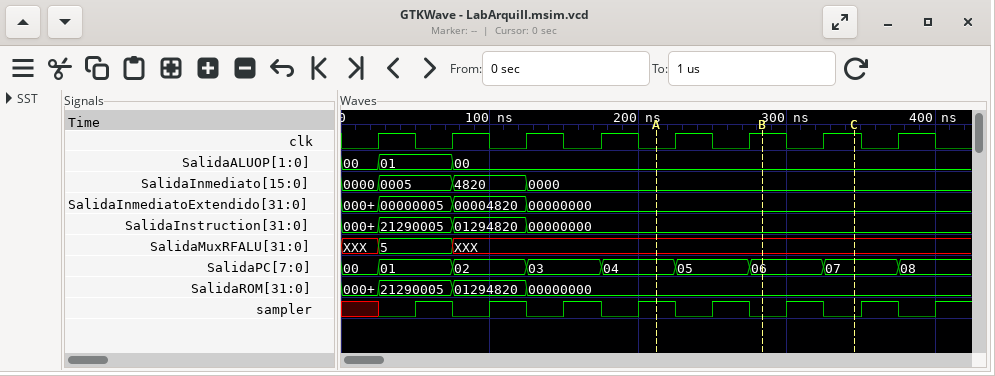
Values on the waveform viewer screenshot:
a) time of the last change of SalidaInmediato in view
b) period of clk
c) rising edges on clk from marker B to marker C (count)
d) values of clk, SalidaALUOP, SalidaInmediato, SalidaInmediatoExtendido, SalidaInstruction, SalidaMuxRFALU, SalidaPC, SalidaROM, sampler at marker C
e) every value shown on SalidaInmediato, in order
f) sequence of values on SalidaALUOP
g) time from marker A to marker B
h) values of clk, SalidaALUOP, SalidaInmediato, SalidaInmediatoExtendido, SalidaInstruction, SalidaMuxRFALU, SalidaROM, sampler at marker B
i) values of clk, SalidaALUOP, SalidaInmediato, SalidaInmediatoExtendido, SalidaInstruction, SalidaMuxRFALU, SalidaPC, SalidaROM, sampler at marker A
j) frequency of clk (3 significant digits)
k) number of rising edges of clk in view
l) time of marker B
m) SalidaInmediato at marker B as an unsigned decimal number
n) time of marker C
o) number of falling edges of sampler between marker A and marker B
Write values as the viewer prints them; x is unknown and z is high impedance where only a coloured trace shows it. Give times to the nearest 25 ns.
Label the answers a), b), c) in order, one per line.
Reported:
a) 125 ns
b) 50 ns
c) 1
d) clk=1, SalidaALUOP=00, SalidaInmediato=0000, SalidaInmediatoExtendido=00000000, SalidaInstruction=00000000, SalidaMuxRFALU=XXX, SalidaPC=07, SalidaROM=00000000, sampler=0
e) 0000, 0005, 4820, 0000
f) 00, 01, 00
g) 75 ns
h) clk=1, SalidaALUOP=00, SalidaInmediato=0000, SalidaInmediatoExtendido=00000000, SalidaInstruction=00000000, SalidaMuxRFALU=XXX, SalidaROM=00000000, sampler=0
i) clk=0, SalidaALUOP=00, SalidaInmediato=0000, SalidaInmediatoExtendido=00000000, SalidaInstruction=00000000, SalidaMuxRFALU=XXX, SalidaPC=04, SalidaROM=00000000, sampler=1
j) 20.0 MHz
k) 8
l) 275 ns
m) 0
n) 350 ns
o) 2
